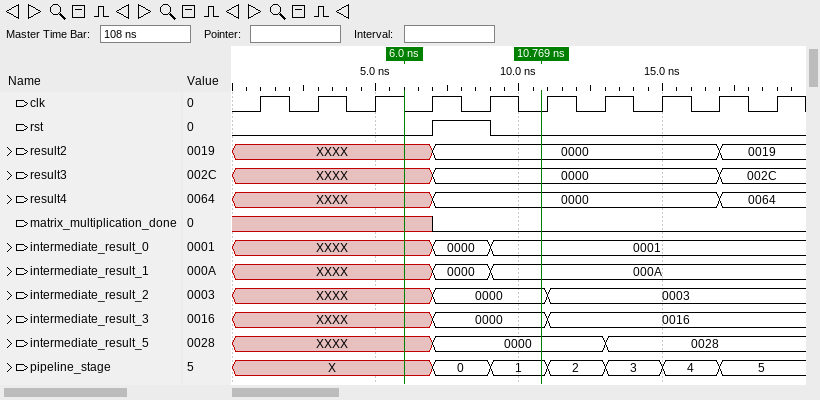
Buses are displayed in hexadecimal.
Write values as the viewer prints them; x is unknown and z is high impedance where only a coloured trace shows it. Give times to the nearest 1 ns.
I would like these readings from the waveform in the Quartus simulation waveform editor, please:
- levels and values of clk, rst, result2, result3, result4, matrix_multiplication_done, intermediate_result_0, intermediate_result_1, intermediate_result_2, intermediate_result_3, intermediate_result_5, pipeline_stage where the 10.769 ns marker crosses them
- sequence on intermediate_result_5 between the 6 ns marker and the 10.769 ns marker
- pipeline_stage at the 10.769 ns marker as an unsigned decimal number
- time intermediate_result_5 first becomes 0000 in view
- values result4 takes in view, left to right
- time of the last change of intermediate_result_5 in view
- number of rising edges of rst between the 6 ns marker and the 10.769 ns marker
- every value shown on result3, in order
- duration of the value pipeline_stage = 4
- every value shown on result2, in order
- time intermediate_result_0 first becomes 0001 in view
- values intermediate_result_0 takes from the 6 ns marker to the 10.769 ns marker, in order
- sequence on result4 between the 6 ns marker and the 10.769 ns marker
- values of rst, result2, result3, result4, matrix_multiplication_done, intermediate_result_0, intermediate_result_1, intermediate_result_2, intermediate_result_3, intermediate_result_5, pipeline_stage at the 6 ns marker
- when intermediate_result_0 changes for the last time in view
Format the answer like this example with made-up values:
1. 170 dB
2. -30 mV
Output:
1. clk=0, rst=0, result2=0000, result3=0000, result4=0000, matrix_multiplication_done=0, intermediate_result_0=0001, intermediate_result_1=000A, intermediate_result_2=0000, intermediate_result_3=0000, intermediate_result_5=0000, pipeline_stage=1
2. XXXX, 0000
3. 1
4. 7 ns
5. XXXX, 0000, 0064
6. 13 ns
7. 1
8. XXXX, 0000, 002C
9. 2 ns
10. XXXX, 0000, 0019
11. 9 ns
12. XXXX, 0000, 0001
13. XXXX, 0000
14. rst=0, result2=XXXX, result3=XXXX, result4=XXXX, matrix_multiplication_done=x, intermediate_result_0=XXXX, intermediate_result_1=XXXX, intermediate_result_2=XXXX, intermediate_result_3=XXXX, intermediate_result_5=XXXX, pipeline_stage=X
15. 9 ns
